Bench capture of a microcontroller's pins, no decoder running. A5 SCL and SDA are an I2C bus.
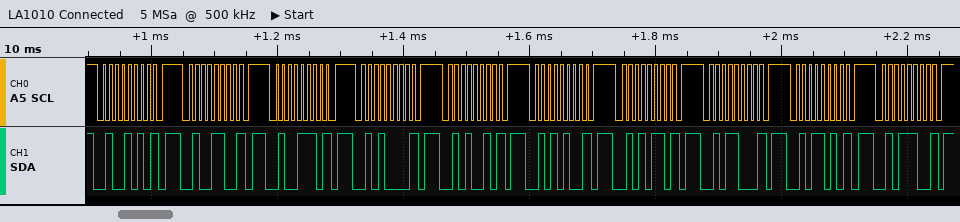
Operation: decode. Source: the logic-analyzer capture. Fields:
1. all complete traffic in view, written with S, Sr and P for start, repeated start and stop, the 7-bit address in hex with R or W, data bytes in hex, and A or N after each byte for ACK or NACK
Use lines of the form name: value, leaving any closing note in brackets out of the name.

all complete traffic in view, written with S, Sr and P for start, repeated start and stop, the 7-bit address in hex with R or W, data bytes in hex, and A or N after each byte for ACK or NACK: S 25W N P S 26W N P S 27W N P S 28W N P S 29W N P S 2AW N P S 2BW N P S 2CW N P S 2DW N P S 2EW N P
